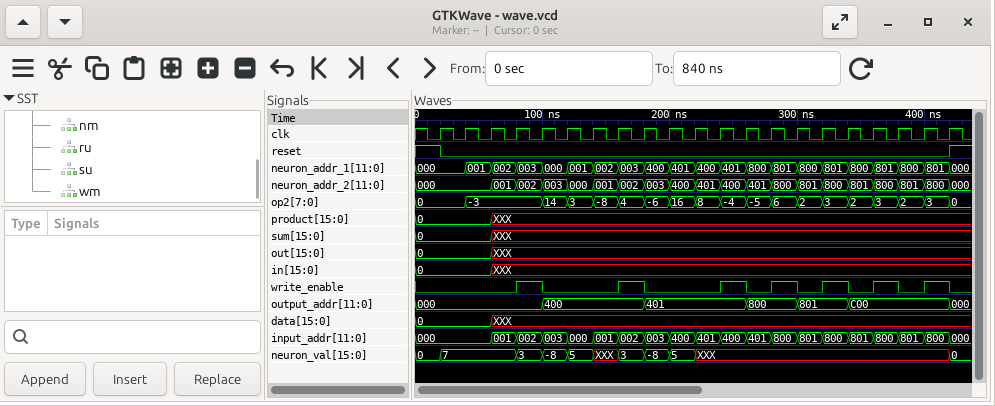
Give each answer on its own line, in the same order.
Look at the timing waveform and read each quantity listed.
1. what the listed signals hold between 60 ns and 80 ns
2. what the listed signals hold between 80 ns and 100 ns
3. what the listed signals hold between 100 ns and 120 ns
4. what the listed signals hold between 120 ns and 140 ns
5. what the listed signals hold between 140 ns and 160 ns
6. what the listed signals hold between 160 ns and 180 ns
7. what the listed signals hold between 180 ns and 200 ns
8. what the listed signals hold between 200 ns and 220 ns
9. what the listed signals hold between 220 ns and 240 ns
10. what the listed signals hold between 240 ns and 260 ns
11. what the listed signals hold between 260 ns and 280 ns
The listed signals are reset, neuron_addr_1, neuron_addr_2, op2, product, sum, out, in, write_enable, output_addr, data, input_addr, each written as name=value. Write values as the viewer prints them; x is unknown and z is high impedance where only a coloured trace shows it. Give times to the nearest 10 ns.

reset=0, neuron_addr_1=002, neuron_addr_2=001, op2=-3, product=XXX, sum=XXX, out=XXX, in=XXX, write_enable=0, output_addr=000, data=XXX, input_addr=001
reset=0, neuron_addr_1=003, neuron_addr_2=002, op2=-3, product=XXX, sum=XXX, out=XXX, in=XXX, write_enable=1, output_addr=000, data=XXX, input_addr=002
reset=0, neuron_addr_1=000, neuron_addr_2=003, op2=14, product=XXX, sum=XXX, out=XXX, in=XXX, write_enable=0, output_addr=400, data=XXX, input_addr=003
reset=0, neuron_addr_1=001, neuron_addr_2=000, op2=3, product=XXX, sum=XXX, out=XXX, in=XXX, write_enable=0, output_addr=400, data=XXX, input_addr=000
reset=0, neuron_addr_1=002, neuron_addr_2=001, op2=-8, product=XXX, sum=XXX, out=XXX, in=XXX, write_enable=0, output_addr=400, data=XXX, input_addr=001
reset=0, neuron_addr_1=003, neuron_addr_2=002, op2=4, product=XXX, sum=XXX, out=XXX, in=XXX, write_enable=1, output_addr=400, data=XXX, input_addr=002
reset=0, neuron_addr_1=400, neuron_addr_2=003, op2=-6, product=XXX, sum=XXX, out=XXX, in=XXX, write_enable=0, output_addr=401, data=XXX, input_addr=003
reset=0, neuron_addr_1=401, neuron_addr_2=400, op2=16, product=XXX, sum=XXX, out=XXX, in=XXX, write_enable=0, output_addr=401, data=XXX, input_addr=400
reset=0, neuron_addr_1=400, neuron_addr_2=401, op2=8, product=XXX, sum=XXX, out=XXX, in=XXX, write_enable=0, output_addr=401, data=XXX, input_addr=401
reset=0, neuron_addr_1=401, neuron_addr_2=400, op2=-4, product=XXX, sum=XXX, out=XXX, in=XXX, write_enable=1, output_addr=401, data=XXX, input_addr=400
reset=0, neuron_addr_1=800, neuron_addr_2=401, op2=-5, product=XXX, sum=XXX, out=XXX, in=XXX, write_enable=0, output_addr=800, data=XXX, input_addr=401
